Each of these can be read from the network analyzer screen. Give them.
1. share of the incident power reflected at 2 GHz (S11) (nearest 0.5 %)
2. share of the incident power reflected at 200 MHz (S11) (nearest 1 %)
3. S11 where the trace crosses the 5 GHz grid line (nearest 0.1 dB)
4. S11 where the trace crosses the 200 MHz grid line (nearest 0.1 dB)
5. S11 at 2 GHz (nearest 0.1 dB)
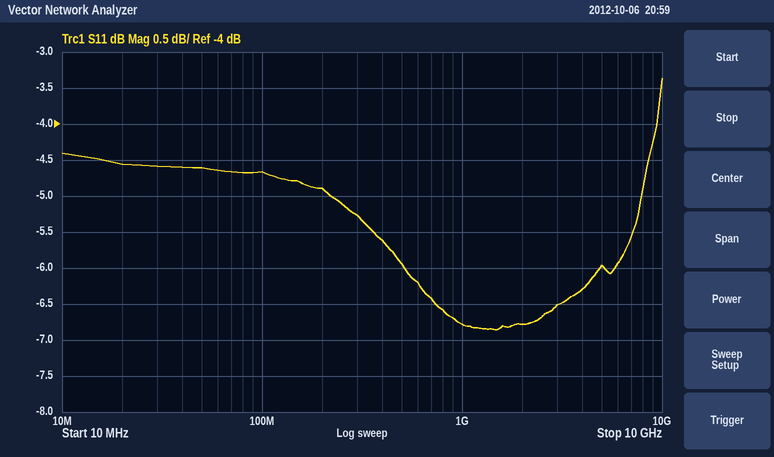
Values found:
21.0 %
32 %
-6.0 dB
-4.9 dB
-6.8 dB
